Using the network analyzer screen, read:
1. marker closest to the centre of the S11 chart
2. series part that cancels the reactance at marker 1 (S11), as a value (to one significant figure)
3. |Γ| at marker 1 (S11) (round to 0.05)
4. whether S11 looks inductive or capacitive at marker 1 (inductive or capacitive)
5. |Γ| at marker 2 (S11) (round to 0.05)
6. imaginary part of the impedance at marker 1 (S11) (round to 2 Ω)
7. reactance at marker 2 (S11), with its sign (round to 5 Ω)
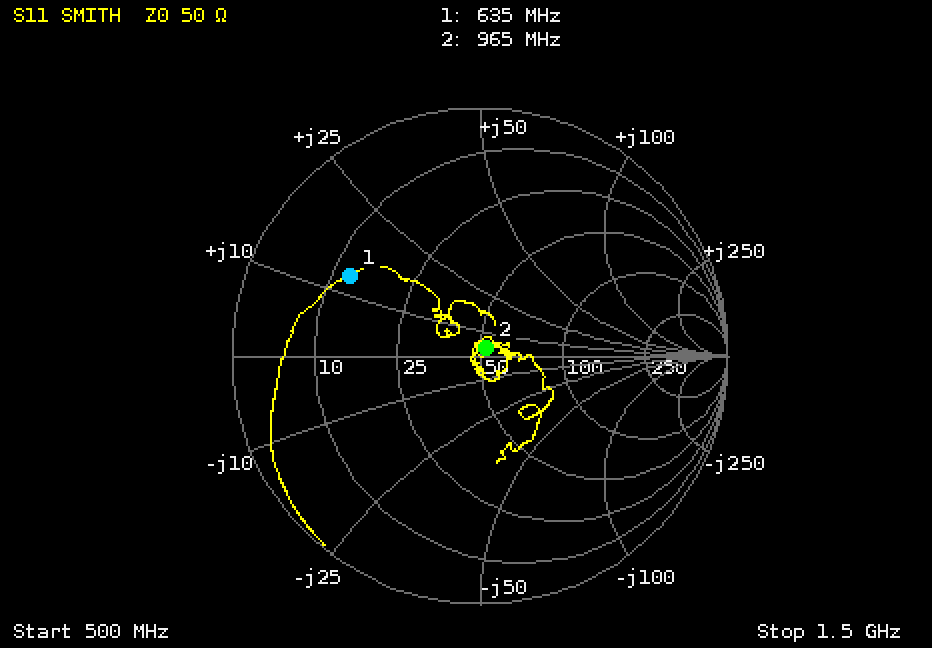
marker 2
20 pF
0.60
inductive
0.05
+14 Ω
+5 Ω
